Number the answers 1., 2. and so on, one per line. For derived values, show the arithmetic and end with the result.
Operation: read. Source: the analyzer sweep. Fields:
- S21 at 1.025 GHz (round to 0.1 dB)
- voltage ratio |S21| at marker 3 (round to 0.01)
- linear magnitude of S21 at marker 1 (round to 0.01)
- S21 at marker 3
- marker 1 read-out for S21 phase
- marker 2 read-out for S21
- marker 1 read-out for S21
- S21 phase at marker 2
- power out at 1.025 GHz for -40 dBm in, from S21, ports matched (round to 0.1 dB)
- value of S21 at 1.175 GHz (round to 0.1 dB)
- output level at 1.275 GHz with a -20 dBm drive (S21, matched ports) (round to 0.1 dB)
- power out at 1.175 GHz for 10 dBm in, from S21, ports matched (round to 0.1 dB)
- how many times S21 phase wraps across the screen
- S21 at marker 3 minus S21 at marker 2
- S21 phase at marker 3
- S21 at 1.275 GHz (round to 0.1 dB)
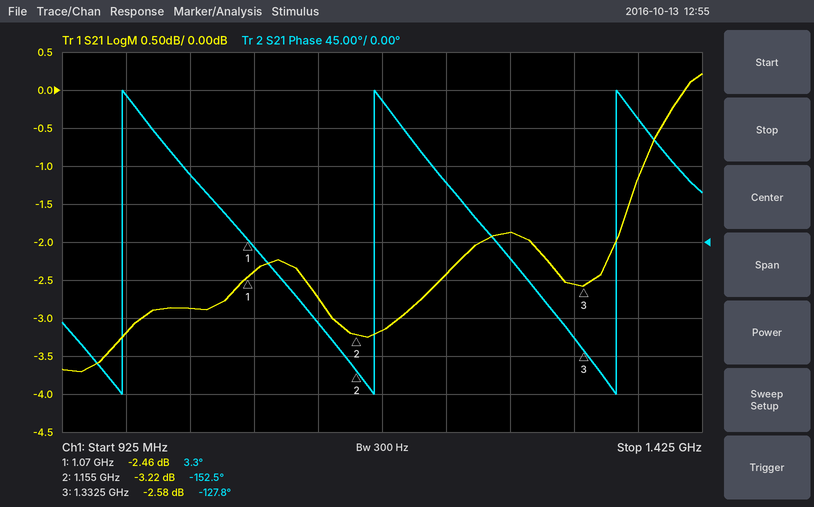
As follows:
1. -2.9 dB
2. 10^(-2.58/20) ≈ 0.74
3. 10^(-2.46/20) ≈ 0.75
4. -2.58 dB
5. 3.3°
6. -3.22 dB
7. -2.46 dB
8. -152.5°
9. -40 dBm + (-2.9 dB) = -42.9 dBm
10. -3.2 dB
11. -20 dBm + (-1.9 dB) = -21.9 dBm
12. 10 dBm + (-3.2 dB) = 6.8 dBm
13. 3
14. -2.58 − (-3.22) = 0.64 dB
15. -127.8°
16. -1.9 dB
